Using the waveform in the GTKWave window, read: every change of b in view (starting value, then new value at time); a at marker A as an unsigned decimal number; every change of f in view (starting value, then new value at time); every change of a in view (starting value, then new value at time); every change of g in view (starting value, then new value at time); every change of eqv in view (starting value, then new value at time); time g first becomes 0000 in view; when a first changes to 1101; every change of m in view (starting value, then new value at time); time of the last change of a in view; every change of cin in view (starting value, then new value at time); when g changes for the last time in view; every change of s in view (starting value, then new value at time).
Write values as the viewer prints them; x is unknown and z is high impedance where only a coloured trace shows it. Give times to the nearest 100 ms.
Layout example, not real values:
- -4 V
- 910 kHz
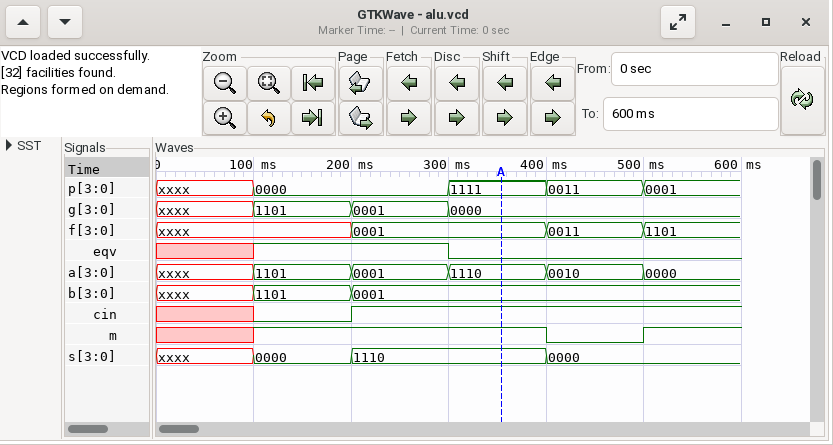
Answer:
- xxxx, 1101 at 100 ms, 0001 at 200 ms
- 14
- xxxx, 0001 at 200 ms, 0011 at 400 ms, 1101 at 500 ms
- xxxx, 1101 at 100 ms, 0001 at 200 ms, 1110 at 300 ms, 0010 at 400 ms, 0000 at 500 ms
- xxxx, 1101 at 100 ms, 0001 at 200 ms, 0000 at 300 ms
- x, 1 at 100 ms, 0 at 300 ms
- 300 ms
- 100 ms
- x, 1 at 100 ms, 0 at 400 ms, 1 at 500 ms
- 500 ms
- x, 0 at 100 ms, 1 at 200 ms
- 300 ms
- xxxx, 0000 at 100 ms, 1110 at 200 ms, 0000 at 400 ms
